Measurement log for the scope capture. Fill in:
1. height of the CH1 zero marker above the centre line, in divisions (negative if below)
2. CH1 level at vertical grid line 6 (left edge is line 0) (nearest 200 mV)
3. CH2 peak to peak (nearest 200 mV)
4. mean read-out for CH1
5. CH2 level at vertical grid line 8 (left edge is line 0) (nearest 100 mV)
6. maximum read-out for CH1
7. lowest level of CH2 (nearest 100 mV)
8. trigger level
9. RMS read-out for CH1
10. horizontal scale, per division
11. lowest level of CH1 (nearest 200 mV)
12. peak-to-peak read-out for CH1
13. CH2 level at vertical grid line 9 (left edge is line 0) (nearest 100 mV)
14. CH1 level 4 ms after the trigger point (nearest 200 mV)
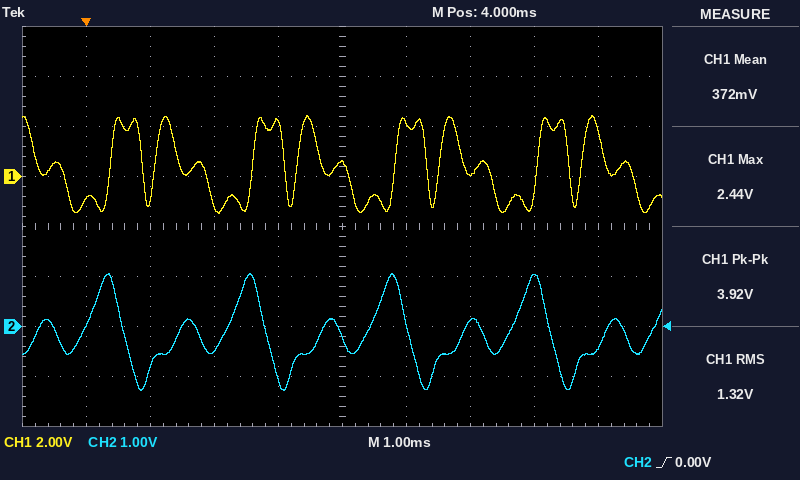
+1.0 div
2.2 V
2.4 V
372 mV
1.0 V
2.44 V
-1.3 V
0.00 V
1.32 V
1 ms
-1.4 V
3.92 V
-400 mV
600 mV
